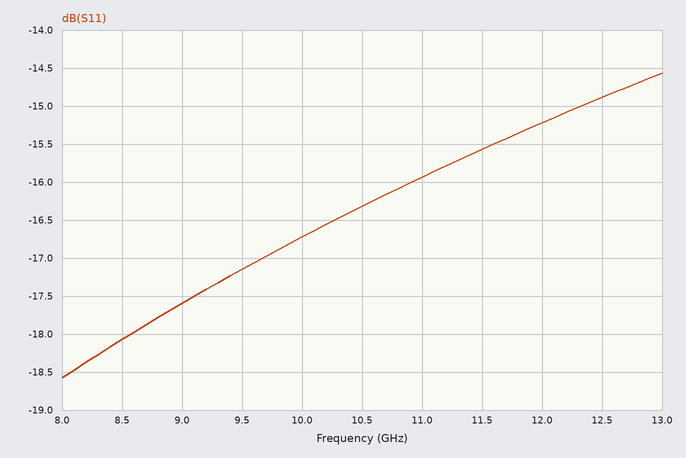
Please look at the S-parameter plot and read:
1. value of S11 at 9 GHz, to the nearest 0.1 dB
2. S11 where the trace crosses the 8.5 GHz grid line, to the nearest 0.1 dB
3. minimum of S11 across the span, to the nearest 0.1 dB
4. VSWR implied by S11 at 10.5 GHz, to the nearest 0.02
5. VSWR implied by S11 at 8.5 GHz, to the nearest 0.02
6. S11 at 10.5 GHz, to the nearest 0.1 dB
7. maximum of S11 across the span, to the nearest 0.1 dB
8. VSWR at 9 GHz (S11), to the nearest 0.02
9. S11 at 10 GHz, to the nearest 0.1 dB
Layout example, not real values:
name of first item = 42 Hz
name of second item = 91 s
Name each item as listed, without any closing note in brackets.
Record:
value of S11 at 9 GHz, to the nearest 0.1 dB = -17.6 dB
S11 where the trace crosses the 8.5 GHz grid line, to the nearest 0.1 dB = -18.1 dB
minimum of S11 across the span, to the nearest 0.1 dB = -18.6 dB
VSWR implied by S11 at 10.5 GHz, to the nearest 0.02 = 1.36
VSWR implied by S11 at 8.5 GHz, to the nearest 0.02 = 1.28
S11 at 10.5 GHz, to the nearest 0.1 dB = -16.3 dB
maximum of S11 across the span, to the nearest 0.1 dB = -14.6 dB
VSWR at 9 GHz (S11), to the nearest 0.02 = 1.30
S11 at 10 GHz, to the nearest 0.1 dB = -16.7 dB
